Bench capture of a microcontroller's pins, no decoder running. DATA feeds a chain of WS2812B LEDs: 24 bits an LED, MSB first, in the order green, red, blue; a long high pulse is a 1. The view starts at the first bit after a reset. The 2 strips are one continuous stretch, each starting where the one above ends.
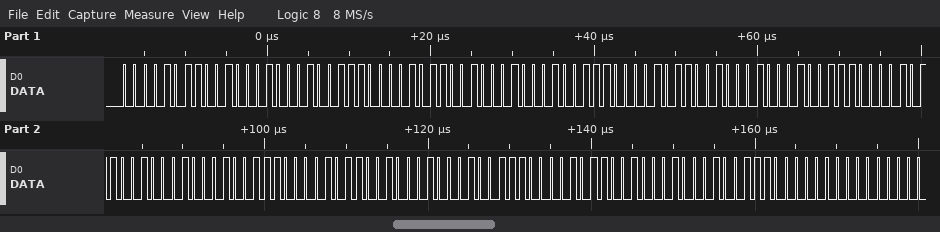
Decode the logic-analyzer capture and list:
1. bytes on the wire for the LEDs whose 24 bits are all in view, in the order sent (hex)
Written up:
0B 22 27 0B 22 27 0B 22 27 0B 22 27 0B 22 27 0B 22 27
